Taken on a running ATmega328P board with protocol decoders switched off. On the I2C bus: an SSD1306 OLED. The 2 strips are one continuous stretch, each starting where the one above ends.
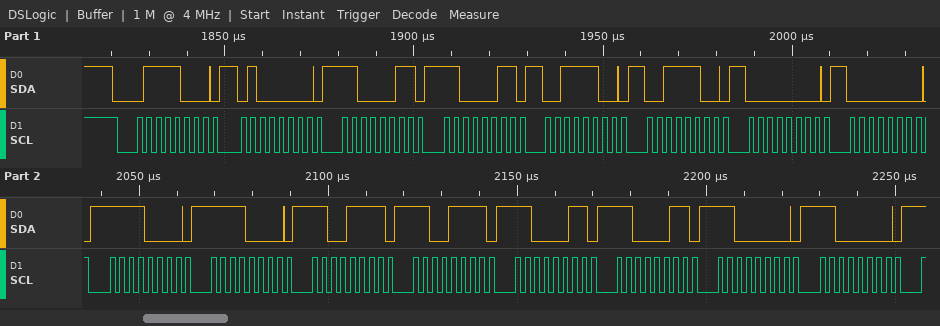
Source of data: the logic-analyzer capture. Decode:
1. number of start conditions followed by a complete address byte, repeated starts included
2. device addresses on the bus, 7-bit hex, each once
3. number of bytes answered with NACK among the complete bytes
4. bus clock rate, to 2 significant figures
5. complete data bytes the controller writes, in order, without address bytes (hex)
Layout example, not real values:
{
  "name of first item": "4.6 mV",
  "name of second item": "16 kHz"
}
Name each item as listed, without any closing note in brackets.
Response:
{
  "number of start conditions followed by a complete address byte, repeated starts included": "1",
  "device addresses on the bus, 7-bit hex, each once": "0x3C",
  "number of bytes answered with NACK among the complete bytes": "0",
  "bus clock rate, to 2 significant figures": "400 kHz",
  "complete data bytes the controller writes, in order, without address bytes": "40 C3 C3 3C 3C 00 00 F0 F0 CF CF C3 C3 C0 C0"
}
